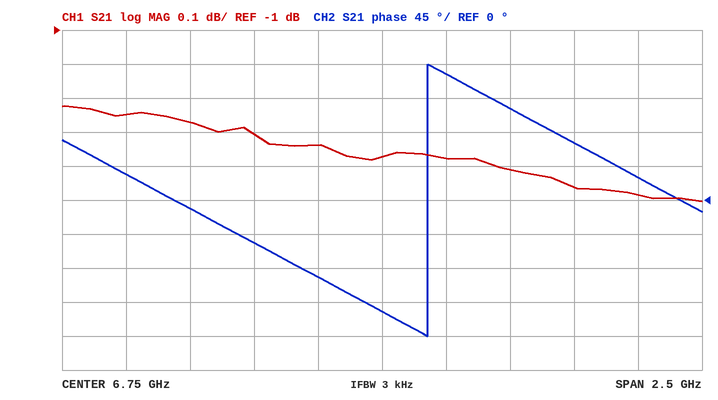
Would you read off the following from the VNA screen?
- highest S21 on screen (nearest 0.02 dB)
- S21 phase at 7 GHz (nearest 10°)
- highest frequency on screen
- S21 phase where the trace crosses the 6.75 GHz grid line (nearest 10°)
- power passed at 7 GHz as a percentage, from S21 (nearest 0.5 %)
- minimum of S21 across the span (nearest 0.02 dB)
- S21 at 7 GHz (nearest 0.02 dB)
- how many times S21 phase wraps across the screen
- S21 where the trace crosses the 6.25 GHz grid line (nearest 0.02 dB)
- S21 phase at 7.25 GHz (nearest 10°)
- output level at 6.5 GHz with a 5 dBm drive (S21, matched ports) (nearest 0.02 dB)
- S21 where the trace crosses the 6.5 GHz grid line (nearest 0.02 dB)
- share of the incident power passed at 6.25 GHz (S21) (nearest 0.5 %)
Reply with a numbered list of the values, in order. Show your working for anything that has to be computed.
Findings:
1. -1.22 dB
2. 170°
3. 8 GHz
4. -150°
5. 10^(-1.38/10) ≈ 72.8 %, so 73.0 % to the nearest 0.5 %
6. -1.50 dB
7. -1.38 dB
8. 1
9. -1.30 dB
10. 120°
11. 5 dBm + (-1.34 dB) = 3.66 dBm
12. -1.34 dB
13. 10^(-1.3/10) ≈ 74.1 %, so 74.0 % to the nearest 0.5 %
